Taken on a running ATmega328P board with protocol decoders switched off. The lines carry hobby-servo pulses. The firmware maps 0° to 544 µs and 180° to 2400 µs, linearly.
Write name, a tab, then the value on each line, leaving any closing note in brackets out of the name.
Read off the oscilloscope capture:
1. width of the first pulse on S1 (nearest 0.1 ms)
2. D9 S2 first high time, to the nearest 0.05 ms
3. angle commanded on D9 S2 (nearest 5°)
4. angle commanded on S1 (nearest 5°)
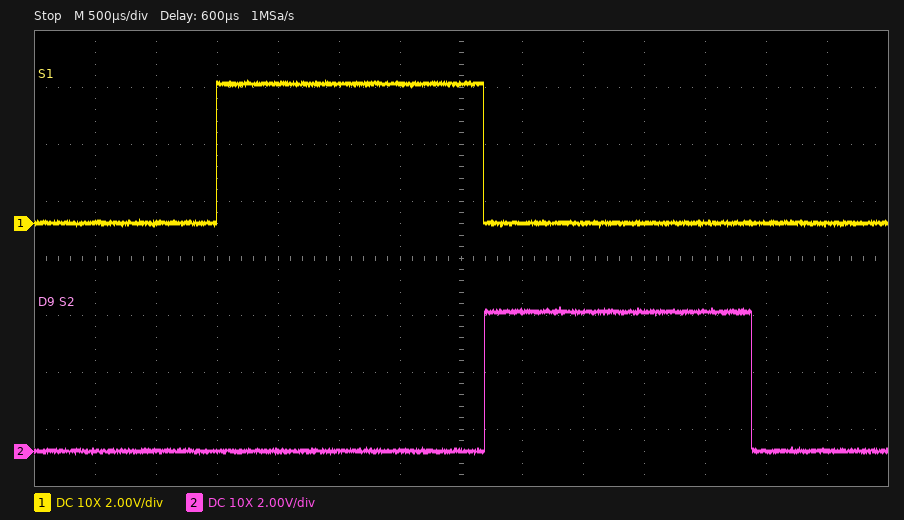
width of the first pulse on S1	2.2 ms
D9 S2 first high time, to the nearest 0.05 ms	2.20 ms
angle commanded on D9 S2	160°
angle commanded on S1	160°
